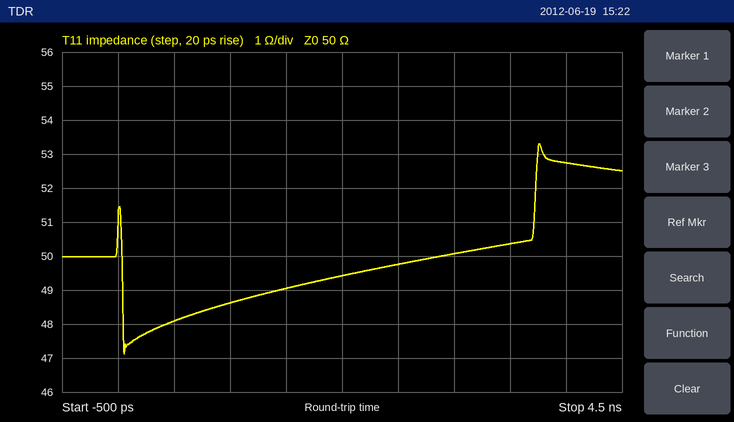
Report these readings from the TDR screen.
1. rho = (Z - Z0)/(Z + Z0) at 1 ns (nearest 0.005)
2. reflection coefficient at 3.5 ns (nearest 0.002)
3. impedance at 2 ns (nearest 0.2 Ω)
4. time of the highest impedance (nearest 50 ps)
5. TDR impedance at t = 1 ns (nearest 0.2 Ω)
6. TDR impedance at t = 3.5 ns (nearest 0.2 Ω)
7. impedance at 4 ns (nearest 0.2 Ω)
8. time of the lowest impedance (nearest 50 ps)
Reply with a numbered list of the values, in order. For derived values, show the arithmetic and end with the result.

1. (48.6 − 50)/(48.6 + 50) ≈ -0.0142, so -0.015 to the nearest 0.005
2. (50.4 − 50)/(50.4 + 50) ≈ +0.004
3. 49.4 Ω
4. 3.75 ns
5. 48.6 Ω
6. 50.4 Ω
7. 52.8 Ω
8. 50 ps
